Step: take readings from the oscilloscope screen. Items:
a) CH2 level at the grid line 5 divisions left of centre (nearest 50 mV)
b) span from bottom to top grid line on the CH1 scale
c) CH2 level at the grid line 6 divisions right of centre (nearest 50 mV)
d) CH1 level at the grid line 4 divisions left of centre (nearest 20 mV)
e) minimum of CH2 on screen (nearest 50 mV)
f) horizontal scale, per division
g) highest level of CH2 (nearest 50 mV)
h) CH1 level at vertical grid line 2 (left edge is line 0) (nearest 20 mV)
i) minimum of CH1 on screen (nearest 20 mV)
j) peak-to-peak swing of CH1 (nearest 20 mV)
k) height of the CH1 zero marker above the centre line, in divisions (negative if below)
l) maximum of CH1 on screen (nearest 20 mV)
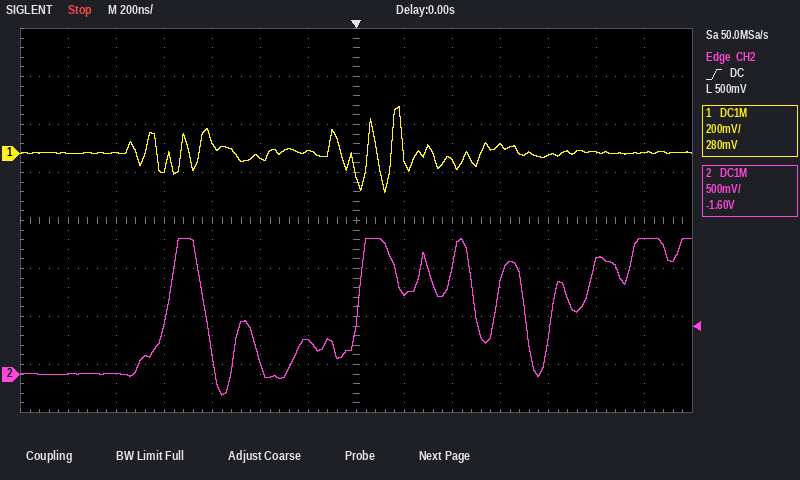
0 mV
1.6 V
1.40 V
-60 mV
-200 mV
200 ns
1.40 V
0 mV
-160 mV
360 mV
+1.4 div
200 mV
